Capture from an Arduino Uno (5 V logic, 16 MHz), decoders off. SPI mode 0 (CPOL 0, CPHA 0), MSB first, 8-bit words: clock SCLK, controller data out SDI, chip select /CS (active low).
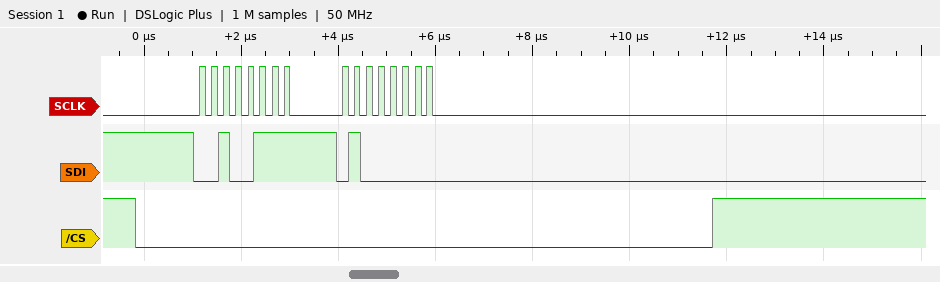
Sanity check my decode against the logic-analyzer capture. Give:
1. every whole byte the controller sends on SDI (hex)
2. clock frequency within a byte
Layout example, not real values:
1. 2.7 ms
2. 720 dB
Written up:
1. 0x27 0x40
2. 4 MHz
